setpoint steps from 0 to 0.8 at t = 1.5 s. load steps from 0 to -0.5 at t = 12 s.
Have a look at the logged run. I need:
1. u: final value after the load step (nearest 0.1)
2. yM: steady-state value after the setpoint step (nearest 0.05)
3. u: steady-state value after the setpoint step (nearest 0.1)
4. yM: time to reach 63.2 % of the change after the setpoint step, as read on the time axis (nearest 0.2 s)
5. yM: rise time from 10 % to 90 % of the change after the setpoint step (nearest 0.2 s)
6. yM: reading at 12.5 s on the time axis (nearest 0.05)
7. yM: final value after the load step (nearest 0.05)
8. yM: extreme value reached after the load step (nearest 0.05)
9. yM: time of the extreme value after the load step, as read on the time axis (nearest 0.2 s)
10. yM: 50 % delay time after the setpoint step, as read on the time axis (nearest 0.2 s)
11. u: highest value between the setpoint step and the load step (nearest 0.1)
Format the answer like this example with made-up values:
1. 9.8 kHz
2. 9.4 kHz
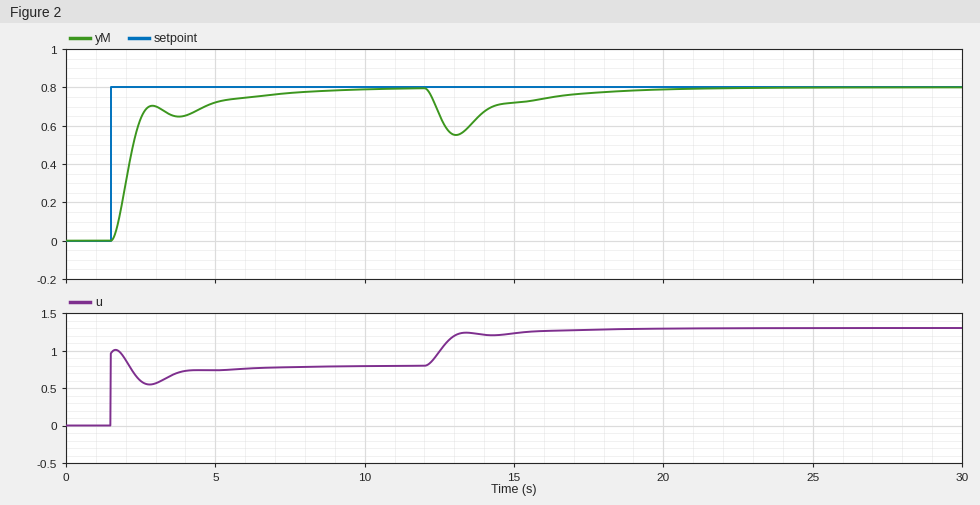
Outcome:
1. 1.3
2. 0.80
3. 0.8
4. 2.2 s
5. 3.2 s
6. 0.65
7. 0.80
8. 0.55
9. 13.0 s
10. 2.2 s
11. 1.0
